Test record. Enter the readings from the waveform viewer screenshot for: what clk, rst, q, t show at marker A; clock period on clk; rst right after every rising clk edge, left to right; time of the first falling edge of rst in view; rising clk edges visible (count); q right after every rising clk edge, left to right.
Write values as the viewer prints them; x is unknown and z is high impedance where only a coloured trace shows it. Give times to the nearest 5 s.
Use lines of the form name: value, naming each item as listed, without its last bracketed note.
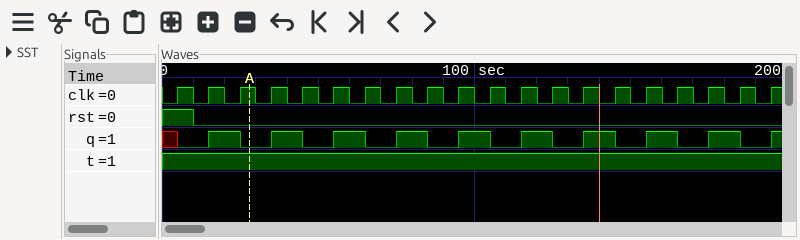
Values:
what clk, rst, q, t show at marker A: clk=1, rst=0, q=0, t=1
clock period on clk: 10 s
rst right after every rising clk edge, left to right: 1 0 0 0 0 0 0 0 0 0 0 0 0 0 0 0 0 0 0 0
time of the first falling edge of rst in view: 10 s
rising clk edges visible: 20
q right after every rising clk edge, left to right: 0 1 0 1 0 1 0 1 0 1 0 1 0 1 0 1 0 1 0 1
